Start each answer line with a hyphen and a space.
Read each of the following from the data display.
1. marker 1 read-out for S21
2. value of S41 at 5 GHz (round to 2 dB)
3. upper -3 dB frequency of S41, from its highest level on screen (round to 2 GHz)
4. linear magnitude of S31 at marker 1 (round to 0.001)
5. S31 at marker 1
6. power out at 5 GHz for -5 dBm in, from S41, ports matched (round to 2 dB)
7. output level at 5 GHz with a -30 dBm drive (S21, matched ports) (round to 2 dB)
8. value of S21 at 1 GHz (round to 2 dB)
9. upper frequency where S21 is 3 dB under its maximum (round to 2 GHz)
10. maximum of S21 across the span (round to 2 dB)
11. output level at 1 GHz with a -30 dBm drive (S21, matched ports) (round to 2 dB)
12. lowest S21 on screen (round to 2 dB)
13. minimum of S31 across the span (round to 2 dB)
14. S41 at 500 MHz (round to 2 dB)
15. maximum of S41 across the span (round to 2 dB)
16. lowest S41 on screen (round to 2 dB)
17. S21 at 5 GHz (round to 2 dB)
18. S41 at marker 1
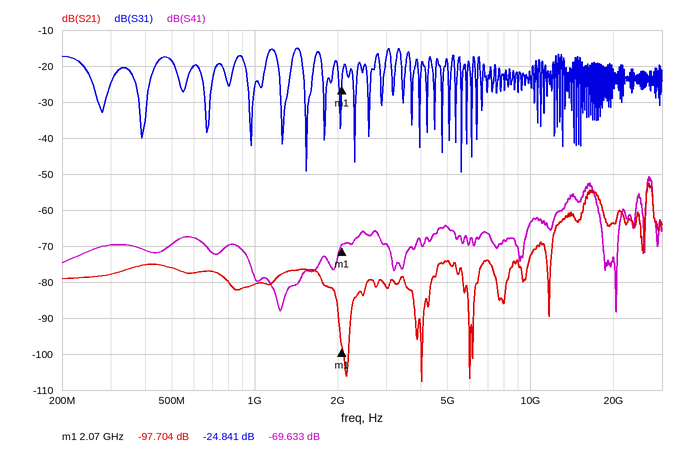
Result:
- -97.704 dB
- -64 dB
- 28 GHz
- 0.057
- -24.841 dB
- -70 dBm
- -104 dBm
- -80 dB
- 28 GHz
- -52 dB
- -110 dBm
- -108 dB
- -50 dB
- -70 dB
- -50 dB
- -88 dB
- -74 dB
- -69.633 dB
